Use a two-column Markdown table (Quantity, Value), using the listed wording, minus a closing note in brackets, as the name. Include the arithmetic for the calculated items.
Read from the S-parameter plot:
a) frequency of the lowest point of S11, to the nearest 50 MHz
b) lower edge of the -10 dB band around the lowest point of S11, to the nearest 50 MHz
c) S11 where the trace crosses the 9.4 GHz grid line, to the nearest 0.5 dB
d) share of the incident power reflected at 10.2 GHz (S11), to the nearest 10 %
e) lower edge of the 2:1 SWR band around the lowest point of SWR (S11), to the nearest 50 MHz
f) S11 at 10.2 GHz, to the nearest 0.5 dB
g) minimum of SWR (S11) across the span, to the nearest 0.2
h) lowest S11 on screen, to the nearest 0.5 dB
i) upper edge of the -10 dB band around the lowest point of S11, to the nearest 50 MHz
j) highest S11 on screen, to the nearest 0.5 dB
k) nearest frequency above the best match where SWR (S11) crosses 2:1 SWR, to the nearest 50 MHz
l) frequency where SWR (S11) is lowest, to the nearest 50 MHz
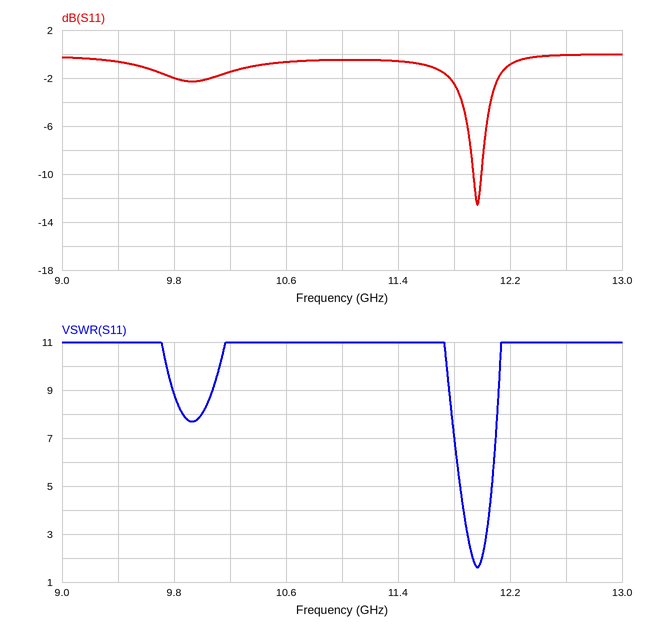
| Quantity | Value |
|---|---|
| frequency of the lowest point of S11, to the nearest 50 MHz | 11.95 GHz |
| lower edge of the -10 dB band around the lowest point of S11, to the nearest 50 MHz | 11.95 GHz |
| S11 where the trace crosses the 9.4 GHz grid line, to the nearest 0.5 dB | -0.5 dB |
| share of the incident power reflected at 10.2 GHz (S11), to the nearest 10 % | 10^(-1.5/10) ≈ 70.8 %, so 70 % to the nearest 10 % |
| lower edge of the 2:1 SWR band around the lowest point of SWR (S11), to the nearest 50 MHz | 11.95 GHz |
| S11 at 10.2 GHz, to the nearest 0.5 dB | -1.5 dB |
| minimum of SWR (S11) across the span, to the nearest 0.2 | 1.6 |
| lowest S11 on screen, to the nearest 0.5 dB | -12.5 dB |
| upper edge of the -10 dB band around the lowest point of S11, to the nearest 50 MHz | 12.00 GHz |
| highest S11 on screen, to the nearest 0.5 dB | 0.0 dB |
| nearest frequency above the best match where SWR (S11) crosses 2:1 SWR, to the nearest 50 MHz | 12.00 GHz |
| frequency where SWR (S11) is lowest, to the nearest 50 MHz | 11.95 GHz |
